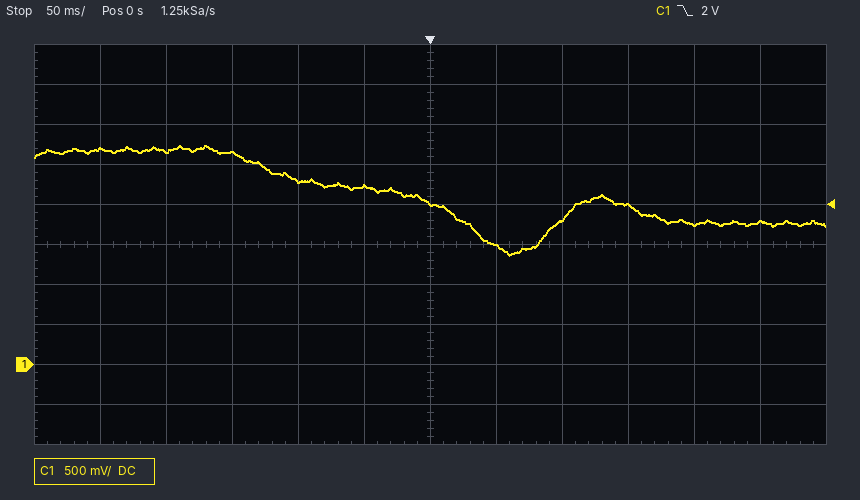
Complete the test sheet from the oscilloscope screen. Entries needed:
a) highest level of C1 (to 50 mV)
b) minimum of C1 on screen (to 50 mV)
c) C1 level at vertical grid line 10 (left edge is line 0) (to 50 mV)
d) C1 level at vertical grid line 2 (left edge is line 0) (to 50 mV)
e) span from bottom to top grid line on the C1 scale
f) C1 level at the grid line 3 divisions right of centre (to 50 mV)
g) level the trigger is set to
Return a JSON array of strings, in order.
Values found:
["2.75 V", "1.35 V", "1.75 V", "2.65 V", "5 V", "2.00 V", "2 V"]
